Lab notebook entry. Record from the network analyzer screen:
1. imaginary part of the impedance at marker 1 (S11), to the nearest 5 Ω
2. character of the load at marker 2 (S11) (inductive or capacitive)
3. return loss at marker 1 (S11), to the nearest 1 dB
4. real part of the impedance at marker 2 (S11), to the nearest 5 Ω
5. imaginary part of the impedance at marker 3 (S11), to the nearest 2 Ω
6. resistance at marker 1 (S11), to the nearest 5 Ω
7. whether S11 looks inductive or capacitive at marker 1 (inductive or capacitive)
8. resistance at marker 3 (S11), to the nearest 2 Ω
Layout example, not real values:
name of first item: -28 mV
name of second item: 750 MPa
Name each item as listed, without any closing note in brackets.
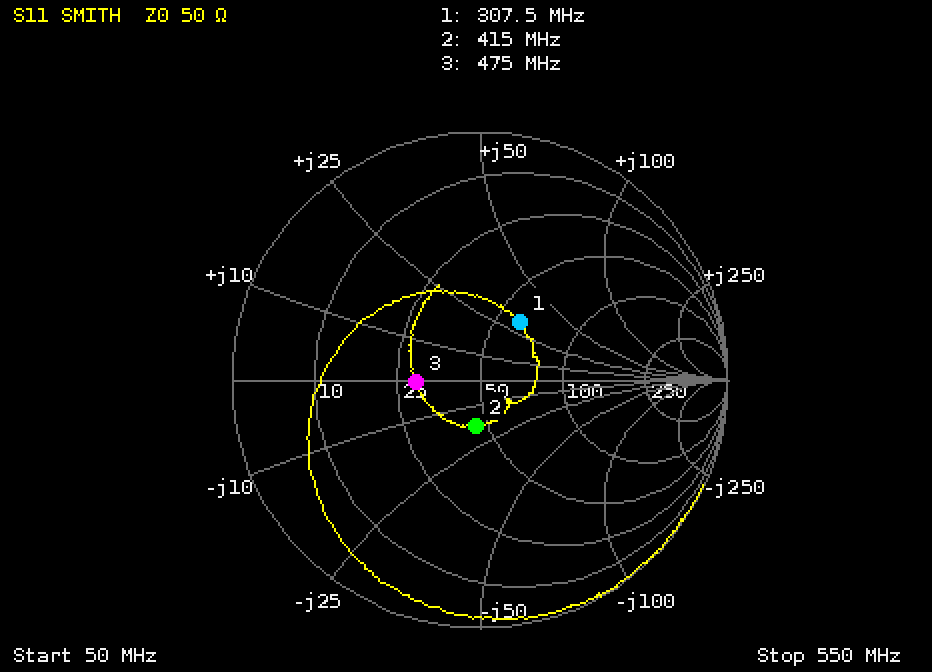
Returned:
imaginary part of the impedance at marker 1 (S11), to the nearest 5 Ω: +30 Ω
character of the load at marker 2 (S11): capacitive
return loss at marker 1 (S11), to the nearest 1 dB: 11 dB
real part of the impedance at marker 2 (S11), to the nearest 5 Ω: 45 Ω
imaginary part of the impedance at marker 3 (S11), to the nearest 2 Ω: 0 Ω
resistance at marker 1 (S11), to the nearest 5 Ω: 60 Ω
whether S11 looks inductive or capacitive at marker 1: inductive
resistance at marker 3 (S11), to the nearest 2 Ω: 30 Ω
